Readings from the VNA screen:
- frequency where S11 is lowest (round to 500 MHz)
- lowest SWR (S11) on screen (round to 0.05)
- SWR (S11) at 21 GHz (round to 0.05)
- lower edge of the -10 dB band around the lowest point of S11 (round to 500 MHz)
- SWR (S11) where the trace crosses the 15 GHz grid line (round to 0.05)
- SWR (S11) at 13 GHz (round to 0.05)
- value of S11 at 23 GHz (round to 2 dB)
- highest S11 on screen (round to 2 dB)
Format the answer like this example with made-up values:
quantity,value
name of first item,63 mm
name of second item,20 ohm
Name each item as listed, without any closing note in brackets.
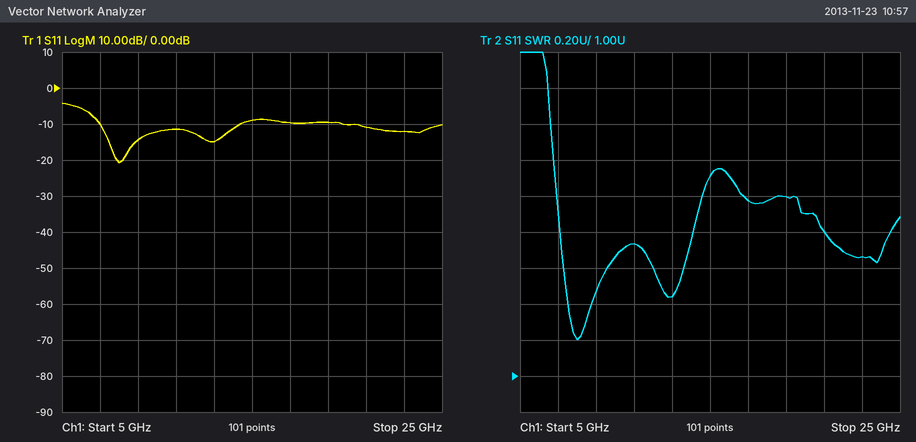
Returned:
quantity,value
frequency where S11 is lowest,8.0 GHz
lowest SWR (S11) on screen,1.20
SWR (S11) at 21 GHz,1.80
lower edge of the -10 dB band around the lowest point of S11,7.0 GHz
SWR (S11) where the trace crosses the 15 GHz grid line,2.10
SWR (S11) at 13 GHz,1.45
value of S11 at 23 GHz,-12 dB
highest S11 on screen,-4 dB
